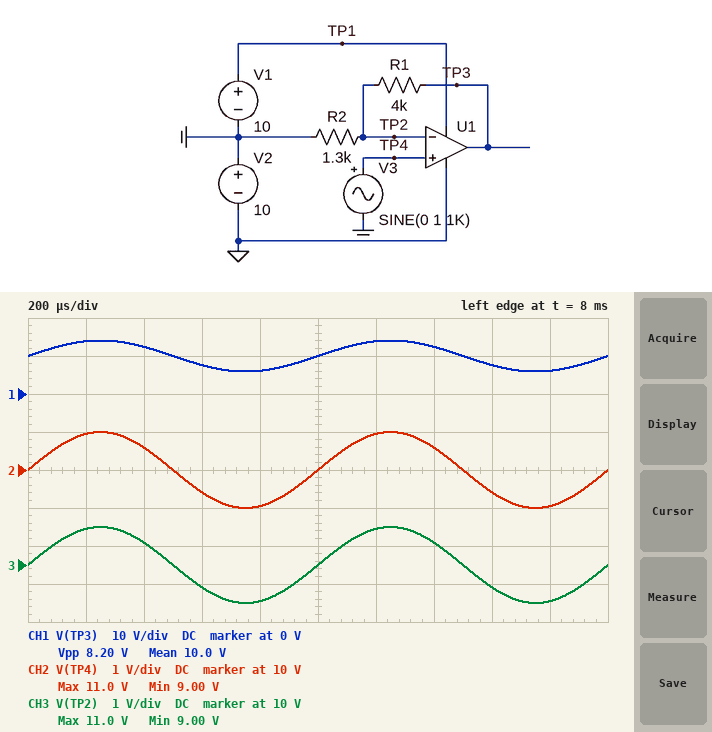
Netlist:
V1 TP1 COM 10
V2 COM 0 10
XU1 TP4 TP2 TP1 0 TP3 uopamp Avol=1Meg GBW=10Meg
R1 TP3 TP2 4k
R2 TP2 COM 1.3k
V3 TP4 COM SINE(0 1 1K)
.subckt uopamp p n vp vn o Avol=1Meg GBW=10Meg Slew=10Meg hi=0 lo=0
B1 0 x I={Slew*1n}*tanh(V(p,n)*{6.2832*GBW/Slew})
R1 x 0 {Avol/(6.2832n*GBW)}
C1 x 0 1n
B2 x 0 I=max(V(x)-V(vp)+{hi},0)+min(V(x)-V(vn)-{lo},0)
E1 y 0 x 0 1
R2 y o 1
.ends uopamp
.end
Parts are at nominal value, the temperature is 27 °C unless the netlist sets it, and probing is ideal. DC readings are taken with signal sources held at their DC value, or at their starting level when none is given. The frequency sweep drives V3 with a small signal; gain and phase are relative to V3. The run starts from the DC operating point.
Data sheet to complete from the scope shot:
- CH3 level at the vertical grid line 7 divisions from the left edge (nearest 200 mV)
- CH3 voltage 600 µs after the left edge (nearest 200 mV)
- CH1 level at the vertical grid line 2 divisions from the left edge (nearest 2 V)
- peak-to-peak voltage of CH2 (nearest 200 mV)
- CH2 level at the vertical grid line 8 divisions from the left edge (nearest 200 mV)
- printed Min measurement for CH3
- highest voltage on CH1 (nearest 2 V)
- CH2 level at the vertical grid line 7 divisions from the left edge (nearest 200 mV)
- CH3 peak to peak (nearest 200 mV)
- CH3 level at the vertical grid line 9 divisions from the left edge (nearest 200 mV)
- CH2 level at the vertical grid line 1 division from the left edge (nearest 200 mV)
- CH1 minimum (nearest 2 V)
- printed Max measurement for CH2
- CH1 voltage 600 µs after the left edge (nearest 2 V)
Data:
10.6 V
9.4 V
12 V
2.0 V
9.4 V
9.00 V
14 V
10.6 V
2.0 V
9.0 V
11.0 V
6 V
11.0 V
8 V
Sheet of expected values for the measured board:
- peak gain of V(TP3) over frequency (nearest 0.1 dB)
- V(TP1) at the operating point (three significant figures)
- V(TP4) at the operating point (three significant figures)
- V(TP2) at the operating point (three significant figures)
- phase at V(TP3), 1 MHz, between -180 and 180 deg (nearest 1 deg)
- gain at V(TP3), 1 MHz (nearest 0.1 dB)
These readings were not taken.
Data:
12.2 dB
20.0 V
10.0 V
10.0 V
-22 deg
11.5 dB
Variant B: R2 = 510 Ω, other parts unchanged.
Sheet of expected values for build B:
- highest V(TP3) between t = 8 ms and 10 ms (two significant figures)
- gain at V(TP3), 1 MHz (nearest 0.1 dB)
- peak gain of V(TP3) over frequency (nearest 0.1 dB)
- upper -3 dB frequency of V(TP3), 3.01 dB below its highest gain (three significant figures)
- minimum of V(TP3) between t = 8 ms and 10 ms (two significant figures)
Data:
19 V
16.4 dB
18.9 dB
1.13 MHz
1.2 V
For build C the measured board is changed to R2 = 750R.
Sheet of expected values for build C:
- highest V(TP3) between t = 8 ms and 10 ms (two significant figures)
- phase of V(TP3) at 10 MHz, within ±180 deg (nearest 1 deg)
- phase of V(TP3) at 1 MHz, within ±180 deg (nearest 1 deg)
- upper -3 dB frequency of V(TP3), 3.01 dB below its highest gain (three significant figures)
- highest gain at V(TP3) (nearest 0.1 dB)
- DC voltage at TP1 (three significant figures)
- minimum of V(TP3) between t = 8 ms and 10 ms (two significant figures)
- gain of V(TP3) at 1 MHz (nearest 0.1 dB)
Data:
16 V
-81 deg
-32 deg
1.58 MHz
16.0 dB
20.0 V
3.7 V
14.6 dB
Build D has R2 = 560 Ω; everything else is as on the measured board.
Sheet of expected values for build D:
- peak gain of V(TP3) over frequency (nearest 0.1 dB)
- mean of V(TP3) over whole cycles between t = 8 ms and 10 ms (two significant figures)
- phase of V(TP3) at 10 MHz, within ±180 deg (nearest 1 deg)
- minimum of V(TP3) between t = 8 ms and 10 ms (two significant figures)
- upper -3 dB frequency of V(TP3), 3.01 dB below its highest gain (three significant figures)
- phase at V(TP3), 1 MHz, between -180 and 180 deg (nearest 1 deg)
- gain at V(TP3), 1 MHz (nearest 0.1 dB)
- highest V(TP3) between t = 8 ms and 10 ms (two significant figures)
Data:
18.2 dB
10 V
-83 deg
1.9 V
1.23 MHz
-39 deg
16.0 dB
18 V
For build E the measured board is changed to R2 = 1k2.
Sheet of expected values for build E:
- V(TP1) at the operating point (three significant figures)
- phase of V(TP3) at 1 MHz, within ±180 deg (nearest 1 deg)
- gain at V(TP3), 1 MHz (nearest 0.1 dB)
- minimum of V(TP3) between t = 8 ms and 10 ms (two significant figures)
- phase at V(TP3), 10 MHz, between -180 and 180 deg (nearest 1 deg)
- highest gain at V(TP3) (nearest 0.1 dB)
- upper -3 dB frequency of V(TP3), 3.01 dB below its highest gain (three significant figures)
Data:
20.0 V
-23 deg
12.0 dB
5.7 V
-77 deg
12.7 dB
2.31 MHz
